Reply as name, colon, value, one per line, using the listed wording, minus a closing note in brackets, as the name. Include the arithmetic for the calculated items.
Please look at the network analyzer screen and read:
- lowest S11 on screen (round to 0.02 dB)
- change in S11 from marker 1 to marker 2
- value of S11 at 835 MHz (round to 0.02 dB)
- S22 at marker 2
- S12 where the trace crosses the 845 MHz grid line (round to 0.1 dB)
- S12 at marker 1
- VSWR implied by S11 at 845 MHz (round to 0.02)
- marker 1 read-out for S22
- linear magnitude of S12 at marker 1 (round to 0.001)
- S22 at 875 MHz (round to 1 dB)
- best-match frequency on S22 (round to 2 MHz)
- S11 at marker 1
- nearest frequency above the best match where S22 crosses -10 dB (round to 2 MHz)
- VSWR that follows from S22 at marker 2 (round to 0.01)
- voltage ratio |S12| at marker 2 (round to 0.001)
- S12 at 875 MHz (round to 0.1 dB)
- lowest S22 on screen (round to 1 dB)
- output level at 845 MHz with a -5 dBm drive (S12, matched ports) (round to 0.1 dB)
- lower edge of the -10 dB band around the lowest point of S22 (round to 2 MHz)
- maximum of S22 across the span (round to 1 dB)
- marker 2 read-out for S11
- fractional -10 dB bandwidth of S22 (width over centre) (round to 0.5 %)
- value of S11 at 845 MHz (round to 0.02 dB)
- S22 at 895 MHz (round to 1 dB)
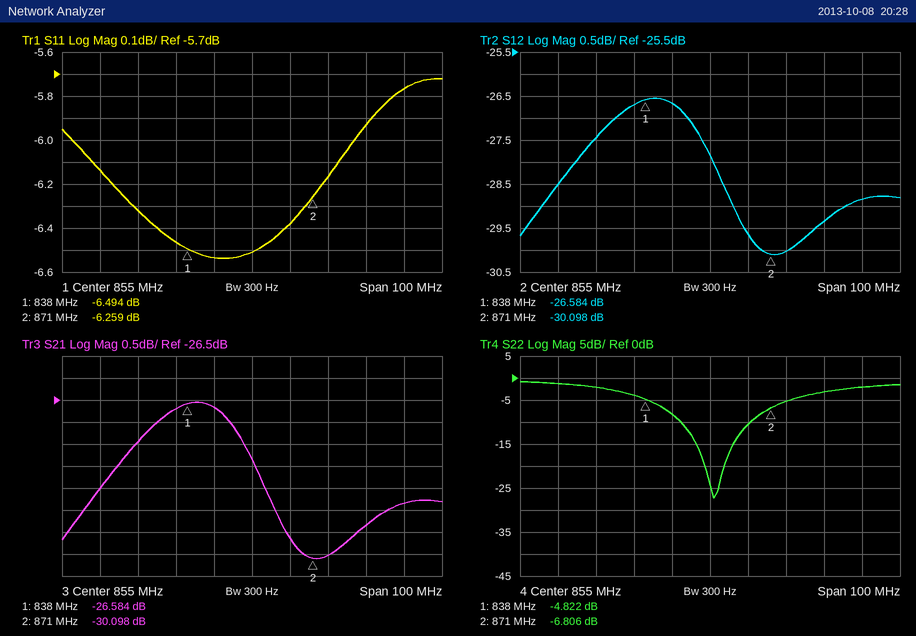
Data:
lowest S11 on screen: -6.54 dB
change in S11 from marker 1 to marker 2: -6.259 − (-6.494) = 0.235 dB
value of S11 at 835 MHz: -6.46 dB
S22 at marker 2: -6.806 dB
S12 where the trace crosses the 845 MHz grid line: -26.7 dB
S12 at marker 1: -26.584 dB
VSWR implied by S11 at 845 MHz: |Γ| = 10^(-6.54/20) = 0.4710; VSWR = (1 + 0.4710)/(1 − 0.4710) ≈ 2.78
marker 1 read-out for S22: -4.822 dB
linear magnitude of S12 at marker 1: 10^(-26.584/20) ≈ 0.047
S22 at 875 MHz: -5 dB
best-match frequency on S22: 856 MHz
S11 at marker 1: -6.494 dB
nearest frequency above the best match where S22 crosses -10 dB: 866 MHz
VSWR that follows from S22 at marker 2: (1 + 0.4568)/(1 − 0.4568) ≈ 2.68
voltage ratio |S12| at marker 2: 10^(-30.098/20) ≈ 0.031
S12 at 875 MHz: -30.0 dB
lowest S22 on screen: -27 dB
output level at 845 MHz with a -5 dBm drive (S12, matched ports): -5 dBm + (-26.7 dB) = -31.7 dBm
lower edge of the -10 dB band around the lowest point of S22: 848 MHz
maximum of S22 across the span: -1 dB
marker 2 read-out for S11: -6.259 dB
fractional -10 dB bandwidth of S22 (width over centre): 18 MHz / 857 MHz ≈ 2.10 %, so 2.0 % to the nearest 0.5 %
value of S11 at 845 MHz: -6.54 dB
S22 at 895 MHz: -2 dB
